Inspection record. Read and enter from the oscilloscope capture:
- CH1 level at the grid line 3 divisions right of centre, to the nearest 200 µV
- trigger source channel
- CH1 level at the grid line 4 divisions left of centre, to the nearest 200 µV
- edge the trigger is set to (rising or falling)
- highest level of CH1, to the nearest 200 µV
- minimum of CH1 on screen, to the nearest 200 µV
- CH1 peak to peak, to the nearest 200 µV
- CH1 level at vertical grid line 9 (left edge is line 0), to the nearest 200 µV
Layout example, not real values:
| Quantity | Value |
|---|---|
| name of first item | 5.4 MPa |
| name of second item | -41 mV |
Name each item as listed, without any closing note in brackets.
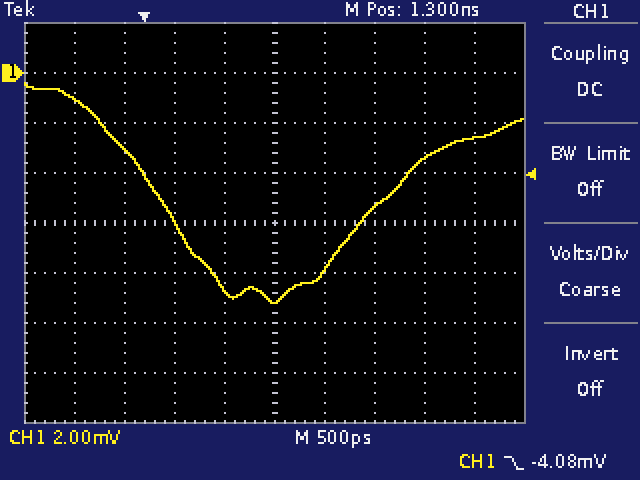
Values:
| Quantity | Value |
|---|---|
| CH1 level at the grid line 3 divisions right of centre, to the nearest 200 µV | -3.4 mV |
| trigger source channel | CH1 |
| CH1 level at the grid line 4 divisions left of centre, to the nearest 200 µV | -1.0 mV |
| edge the trigger is set to | falling |
| highest level of CH1, to the nearest 200 µV | -400 µV |
| minimum of CH1 on screen, to the nearest 200 µV | -9.2 mV |
| CH1 peak to peak, to the nearest 200 µV | 8.8 mV |
| CH1 level at vertical grid line 9 (left edge is line 0), to the nearest 200 µV | -2.6 mV |
